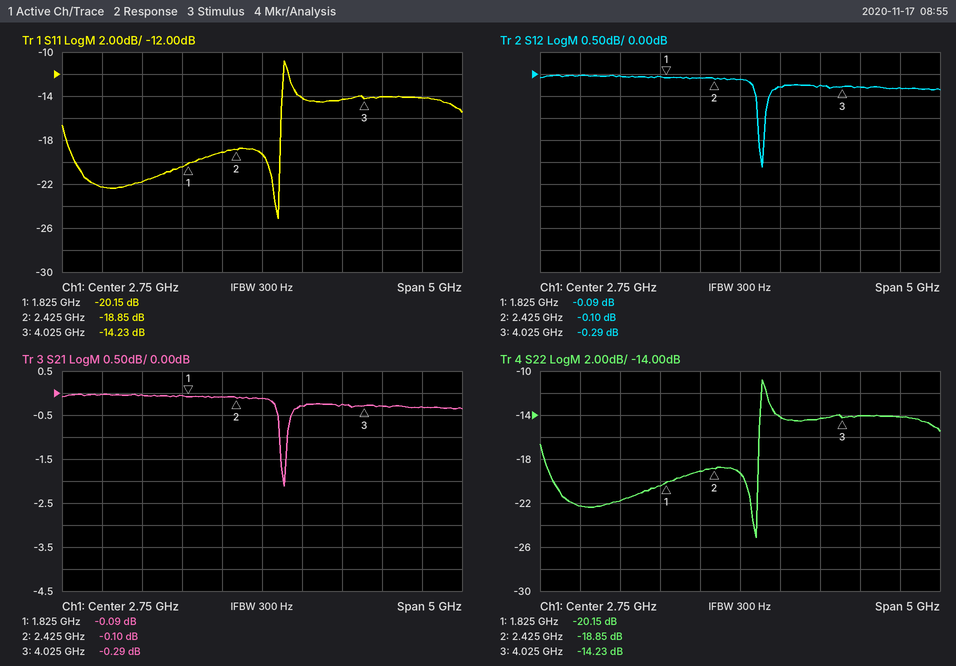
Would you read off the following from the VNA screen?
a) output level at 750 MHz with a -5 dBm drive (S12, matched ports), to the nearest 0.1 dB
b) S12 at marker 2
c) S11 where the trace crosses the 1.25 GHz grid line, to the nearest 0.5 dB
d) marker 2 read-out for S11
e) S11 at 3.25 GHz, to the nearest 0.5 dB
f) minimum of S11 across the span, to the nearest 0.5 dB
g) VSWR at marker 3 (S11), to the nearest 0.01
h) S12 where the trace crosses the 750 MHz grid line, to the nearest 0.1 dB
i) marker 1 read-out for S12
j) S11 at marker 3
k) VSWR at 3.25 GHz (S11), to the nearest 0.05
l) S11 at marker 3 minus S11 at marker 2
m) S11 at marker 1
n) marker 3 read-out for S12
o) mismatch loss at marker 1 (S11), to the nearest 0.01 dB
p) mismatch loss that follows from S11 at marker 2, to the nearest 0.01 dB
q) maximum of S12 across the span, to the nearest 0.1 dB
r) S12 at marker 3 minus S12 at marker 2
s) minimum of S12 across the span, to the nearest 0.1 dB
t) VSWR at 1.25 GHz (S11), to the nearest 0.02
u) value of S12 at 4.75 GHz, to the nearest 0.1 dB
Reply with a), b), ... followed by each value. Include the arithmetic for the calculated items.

a) -5 dBm + (0.0 dB) = -5.0 dBm
b) -0.10 dB
c) -22.0 dB
d) -18.85 dB
e) -14.0 dB
f) -25.0 dB
g) (1 + 0.1943)/(1 − 0.1943) ≈ 1.48
h) 0.0 dB
i) -0.09 dB
j) -14.23 dB
k) |Γ| = 10^(-14/20) = 0.1995; VSWR = (1 + 0.1995)/(1 − 0.1995) ≈ 1.50
l) -14.23 − (-18.85) = 4.62 dB
m) -20.15 dB
n) -0.29 dB
o) −10 log10(1 − 10^(-20.15/10)) ≈ 0.04 dB
p) −10 log10(1 − 10^(-18.85/10)) ≈ 0.06 dB
q) 0.0 dB
r) -0.29 − (-0.1) = -0.19 dB
s) -2.1 dB
t) |Γ| = 10^(-22/20) = 0.0794; VSWR = (1 + 0.0794)/(1 − 0.0794) ≈ 1.17, so 1.18 to the nearest 0.02
u) -0.3 dB
